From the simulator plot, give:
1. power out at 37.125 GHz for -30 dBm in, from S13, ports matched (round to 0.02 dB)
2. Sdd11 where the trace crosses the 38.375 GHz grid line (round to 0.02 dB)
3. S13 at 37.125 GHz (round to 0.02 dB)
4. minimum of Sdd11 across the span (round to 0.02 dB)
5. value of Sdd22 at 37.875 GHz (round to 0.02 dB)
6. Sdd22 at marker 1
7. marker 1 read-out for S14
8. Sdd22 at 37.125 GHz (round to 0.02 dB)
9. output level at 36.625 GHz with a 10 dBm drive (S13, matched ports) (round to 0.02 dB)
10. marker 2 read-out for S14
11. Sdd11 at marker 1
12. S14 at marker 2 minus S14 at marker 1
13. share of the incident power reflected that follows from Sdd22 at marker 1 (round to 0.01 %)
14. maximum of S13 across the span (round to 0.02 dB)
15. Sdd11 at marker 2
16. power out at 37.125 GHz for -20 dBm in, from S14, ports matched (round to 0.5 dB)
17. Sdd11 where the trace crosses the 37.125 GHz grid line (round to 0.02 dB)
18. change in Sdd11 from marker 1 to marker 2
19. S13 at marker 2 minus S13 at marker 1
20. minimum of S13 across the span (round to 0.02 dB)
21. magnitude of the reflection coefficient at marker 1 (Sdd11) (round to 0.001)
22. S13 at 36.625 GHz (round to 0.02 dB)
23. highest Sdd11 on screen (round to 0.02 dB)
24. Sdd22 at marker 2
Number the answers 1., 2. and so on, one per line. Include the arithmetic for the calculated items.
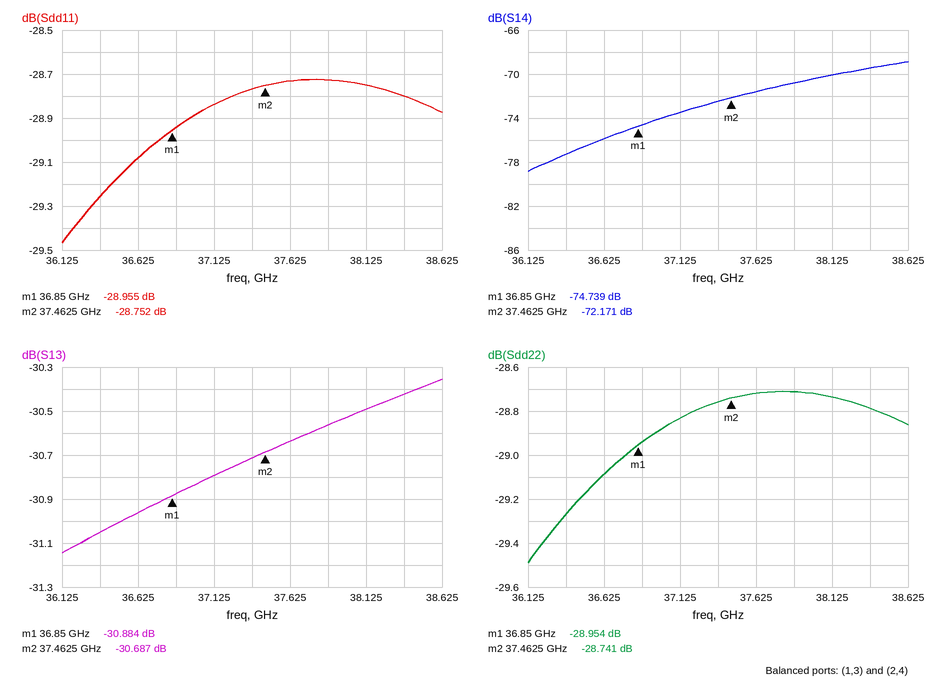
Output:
1. -30 dBm + (-30.80 dB) = -60.80 dBm
2. -28.80 dB
3. -30.80 dB
4. -29.46 dB
5. -28.72 dB
6. -28.954 dB
7. -74.739 dB
8. -28.84 dB
9. 10 dBm + (-30.96 dB) = -20.96 dBm
10. -72.171 dB
11. -28.955 dB
12. -72.171 − (-74.739) = 2.568 dB
13. 10^(-28.954/10) ≈ 0.13 %
14. -30.36 dB
15. -28.752 dB
16. -20 dBm + (-73.5 dB) = -93.5 dBm
17. -28.84 dB
18. -28.752 − (-28.955) = 0.203 dB
19. -30.687 − (-30.884) = 0.197 dB
20. -31.14 dB
21. 10^(-28.955/20) ≈ 0.036
22. -30.96 dB
23. -28.72 dB
24. -28.741 dB
